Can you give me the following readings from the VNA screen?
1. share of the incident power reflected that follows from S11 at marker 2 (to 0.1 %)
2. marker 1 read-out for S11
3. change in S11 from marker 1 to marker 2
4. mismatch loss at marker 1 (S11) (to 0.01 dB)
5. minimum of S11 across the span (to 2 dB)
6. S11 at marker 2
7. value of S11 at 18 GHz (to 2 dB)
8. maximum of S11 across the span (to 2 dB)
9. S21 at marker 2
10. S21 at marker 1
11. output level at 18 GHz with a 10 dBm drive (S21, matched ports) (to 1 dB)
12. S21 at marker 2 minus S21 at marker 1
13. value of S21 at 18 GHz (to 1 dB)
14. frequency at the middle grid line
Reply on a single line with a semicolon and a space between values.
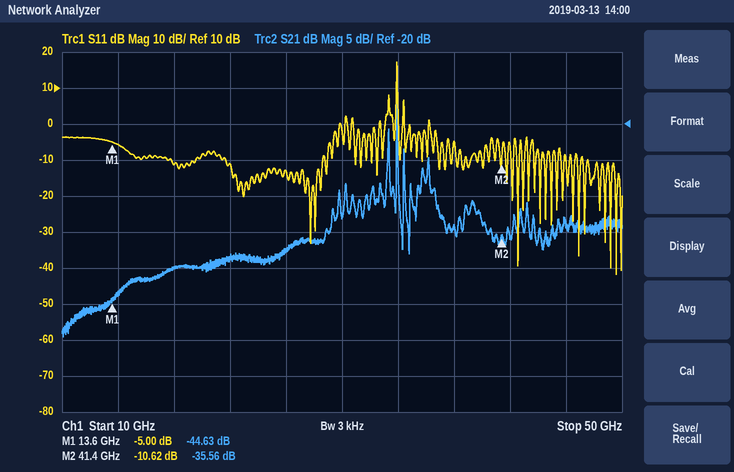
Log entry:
8.7 %; -5.00 dB; -5.62 dB; 1.65 dB; -42 dB; -10.62 dB; -12 dB; 18 dB; -35.56 dB; -44.63 dB; -30 dBm; 9.07 dB; -40 dB; 30 GHz
